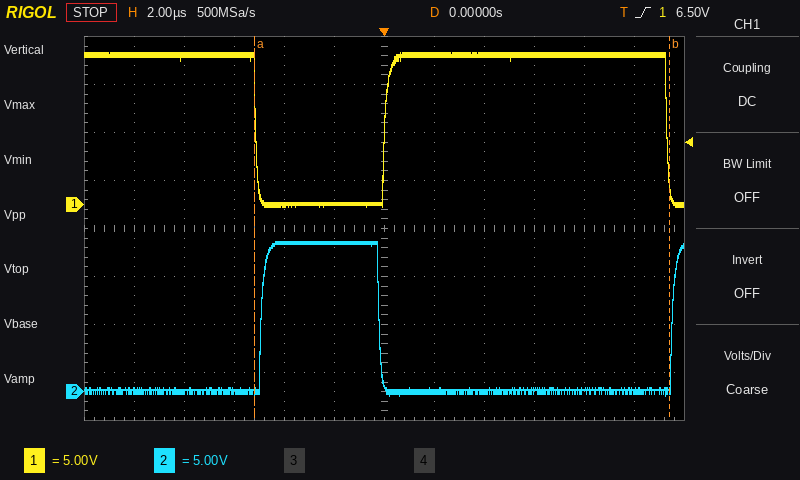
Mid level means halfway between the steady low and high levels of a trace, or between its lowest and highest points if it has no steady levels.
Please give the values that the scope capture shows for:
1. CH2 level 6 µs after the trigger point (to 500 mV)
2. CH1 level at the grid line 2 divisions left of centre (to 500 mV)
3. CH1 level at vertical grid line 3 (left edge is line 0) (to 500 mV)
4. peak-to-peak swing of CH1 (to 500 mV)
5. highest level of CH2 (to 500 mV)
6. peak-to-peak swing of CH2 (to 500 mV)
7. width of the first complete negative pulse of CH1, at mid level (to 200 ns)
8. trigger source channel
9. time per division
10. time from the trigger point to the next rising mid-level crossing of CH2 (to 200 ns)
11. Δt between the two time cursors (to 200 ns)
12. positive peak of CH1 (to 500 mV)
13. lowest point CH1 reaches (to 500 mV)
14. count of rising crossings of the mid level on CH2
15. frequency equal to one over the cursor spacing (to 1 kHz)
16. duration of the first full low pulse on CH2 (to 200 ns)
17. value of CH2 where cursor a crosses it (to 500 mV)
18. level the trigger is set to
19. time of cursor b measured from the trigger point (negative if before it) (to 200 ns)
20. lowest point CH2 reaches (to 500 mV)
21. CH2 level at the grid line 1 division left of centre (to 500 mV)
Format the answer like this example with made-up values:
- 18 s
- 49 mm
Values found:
- 0.0 V
- 0.0 V
- 15.5 V
- 16.0 V
- 15.5 V
- 16.0 V
- 5.2 µs
- CH1
- 2 µs
- 11.6 µs
- 16.6 µs
- 16.0 V
- 0.0 V
- 2
- 60 kHz
- 11.8 µs
- 0.0 V
- 6.50 V
- +11.4 µs
- -500 mV
- 15.5 V
